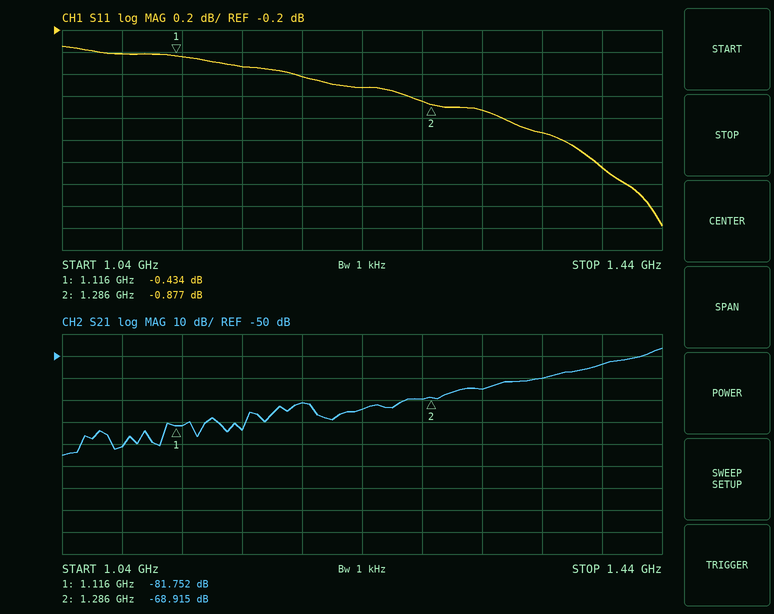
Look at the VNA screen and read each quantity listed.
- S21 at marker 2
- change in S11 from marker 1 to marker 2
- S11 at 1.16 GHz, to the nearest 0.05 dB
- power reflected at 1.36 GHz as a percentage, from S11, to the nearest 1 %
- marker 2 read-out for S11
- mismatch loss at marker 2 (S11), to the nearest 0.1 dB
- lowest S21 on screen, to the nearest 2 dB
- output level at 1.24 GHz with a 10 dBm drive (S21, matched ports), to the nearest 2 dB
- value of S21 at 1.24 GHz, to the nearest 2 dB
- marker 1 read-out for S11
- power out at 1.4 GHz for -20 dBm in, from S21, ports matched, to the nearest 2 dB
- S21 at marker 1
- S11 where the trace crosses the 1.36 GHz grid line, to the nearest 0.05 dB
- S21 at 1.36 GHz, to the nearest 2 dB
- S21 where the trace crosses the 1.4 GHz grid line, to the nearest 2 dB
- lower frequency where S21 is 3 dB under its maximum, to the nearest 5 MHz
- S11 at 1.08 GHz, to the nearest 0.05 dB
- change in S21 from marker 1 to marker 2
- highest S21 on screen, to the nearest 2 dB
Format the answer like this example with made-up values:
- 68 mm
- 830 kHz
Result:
- -68.915 dB
- -0.443 dB
- -0.55 dB
- 77 %
- -0.877 dB
- 7.4 dB
- -96 dB
- -64 dBm
- -74 dB
- -0.434 dB
- -74 dBm
- -81.752 dB
- -1.15 dB
- -60 dB
- -54 dB
- 1.430 GHz
- -0.40 dB
- 12.837 dB
- -46 dB
